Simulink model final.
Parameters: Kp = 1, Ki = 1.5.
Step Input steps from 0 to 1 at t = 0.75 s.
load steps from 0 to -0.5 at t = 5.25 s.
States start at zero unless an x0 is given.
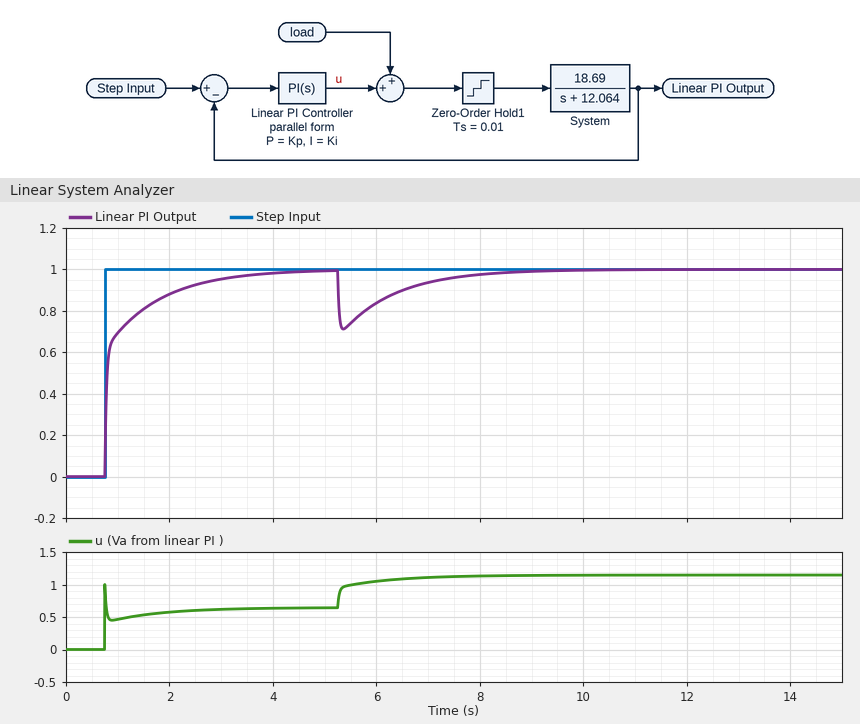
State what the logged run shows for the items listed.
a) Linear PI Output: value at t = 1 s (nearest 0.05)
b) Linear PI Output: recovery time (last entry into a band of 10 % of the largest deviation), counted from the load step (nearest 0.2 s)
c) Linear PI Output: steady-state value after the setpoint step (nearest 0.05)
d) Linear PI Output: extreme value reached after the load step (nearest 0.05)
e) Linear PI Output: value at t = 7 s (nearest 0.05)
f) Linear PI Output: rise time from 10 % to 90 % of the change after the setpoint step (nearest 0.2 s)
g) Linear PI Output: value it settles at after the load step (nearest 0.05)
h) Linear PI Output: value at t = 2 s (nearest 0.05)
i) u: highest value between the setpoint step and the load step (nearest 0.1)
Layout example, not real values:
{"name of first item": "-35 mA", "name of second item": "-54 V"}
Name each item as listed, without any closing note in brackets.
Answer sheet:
{"Linear PI Output: value at t = 1 s": "0.70", "Linear PI Output: recovery time (last entry into a band of 10 % of the largest deviation), counted from the load step": "2.6 s", "Linear PI Output: steady-state value after the setpoint step": "1.00", "Linear PI Output: extreme value reached after the load step": "0.70", "Linear PI Output: value at t = 7 s": "0.95", "Linear PI Output: rise time from 10 % to 90 % of the change after the setpoint step": "1.4 s", "Linear PI Output: value it settles at after the load step": "1.00", "Linear PI Output: value at t = 2 s": "0.90", "u: highest value between the setpoint step and the load step": "1.0"}
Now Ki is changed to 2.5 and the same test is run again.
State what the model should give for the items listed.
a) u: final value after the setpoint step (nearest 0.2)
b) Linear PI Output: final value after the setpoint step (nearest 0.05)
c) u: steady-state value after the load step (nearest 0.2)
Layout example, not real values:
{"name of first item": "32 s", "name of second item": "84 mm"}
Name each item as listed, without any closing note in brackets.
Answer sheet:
{"u: final value after the setpoint step": "0.6", "Linear PI Output: final value after the setpoint step": "1.00", "u: steady-state value after the load step": "1.2"}
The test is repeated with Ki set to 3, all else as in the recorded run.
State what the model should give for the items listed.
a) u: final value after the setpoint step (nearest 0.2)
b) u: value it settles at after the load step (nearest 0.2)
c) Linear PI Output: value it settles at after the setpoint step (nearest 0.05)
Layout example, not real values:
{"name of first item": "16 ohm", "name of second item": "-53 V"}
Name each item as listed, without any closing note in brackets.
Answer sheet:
{"u: final value after the setpoint step": "0.6", "u: value it settles at after the load step": "1.2", "Linear PI Output: value it settles at after the setpoint step": "1.00"}
